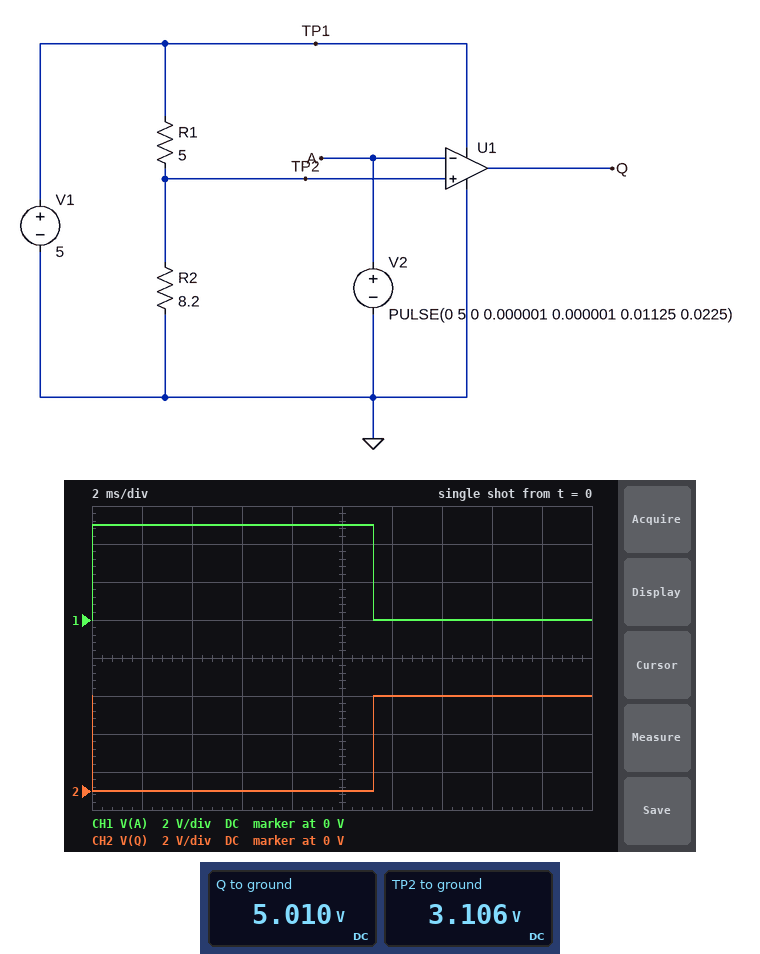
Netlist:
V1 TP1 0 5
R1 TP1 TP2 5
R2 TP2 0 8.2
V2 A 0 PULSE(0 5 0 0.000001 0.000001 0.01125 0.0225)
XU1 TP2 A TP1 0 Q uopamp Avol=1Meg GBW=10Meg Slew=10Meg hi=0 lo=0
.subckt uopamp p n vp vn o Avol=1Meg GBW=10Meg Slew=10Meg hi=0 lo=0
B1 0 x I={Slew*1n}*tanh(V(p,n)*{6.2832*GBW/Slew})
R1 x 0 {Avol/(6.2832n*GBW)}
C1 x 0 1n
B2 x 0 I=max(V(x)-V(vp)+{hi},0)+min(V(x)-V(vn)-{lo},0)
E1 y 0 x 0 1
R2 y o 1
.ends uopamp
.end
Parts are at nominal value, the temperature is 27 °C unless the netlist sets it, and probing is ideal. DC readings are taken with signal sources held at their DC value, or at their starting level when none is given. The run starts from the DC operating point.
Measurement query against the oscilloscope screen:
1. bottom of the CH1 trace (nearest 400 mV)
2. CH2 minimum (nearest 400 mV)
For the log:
0 V
0 V
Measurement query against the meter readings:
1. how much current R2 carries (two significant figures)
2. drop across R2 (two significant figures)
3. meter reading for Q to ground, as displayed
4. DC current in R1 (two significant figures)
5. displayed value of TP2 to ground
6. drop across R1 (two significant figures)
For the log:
380 mA
3.1 V
5.010 V
380 mA
3.106 V
1.9 V
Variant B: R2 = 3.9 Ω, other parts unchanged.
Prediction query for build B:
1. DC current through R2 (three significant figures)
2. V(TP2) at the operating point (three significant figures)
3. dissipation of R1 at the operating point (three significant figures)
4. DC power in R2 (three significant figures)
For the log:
562 mA
2.19 V
1.58 W
1.23 W
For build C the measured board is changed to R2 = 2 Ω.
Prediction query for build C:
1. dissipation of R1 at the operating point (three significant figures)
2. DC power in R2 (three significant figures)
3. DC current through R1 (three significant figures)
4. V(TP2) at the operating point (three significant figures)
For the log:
2.55 W
1.02 W
714 mA
1.43 V
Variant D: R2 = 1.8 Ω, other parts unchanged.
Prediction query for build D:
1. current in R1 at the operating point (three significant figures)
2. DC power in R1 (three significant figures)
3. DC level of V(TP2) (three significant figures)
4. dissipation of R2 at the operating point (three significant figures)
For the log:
735 mA
2.70 W
1.32 V
973 mW
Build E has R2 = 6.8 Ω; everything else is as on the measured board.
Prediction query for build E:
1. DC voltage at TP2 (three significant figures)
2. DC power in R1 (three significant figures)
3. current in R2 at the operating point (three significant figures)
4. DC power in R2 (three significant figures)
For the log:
2.88 V
898 mW
424 mA
1.22 W
